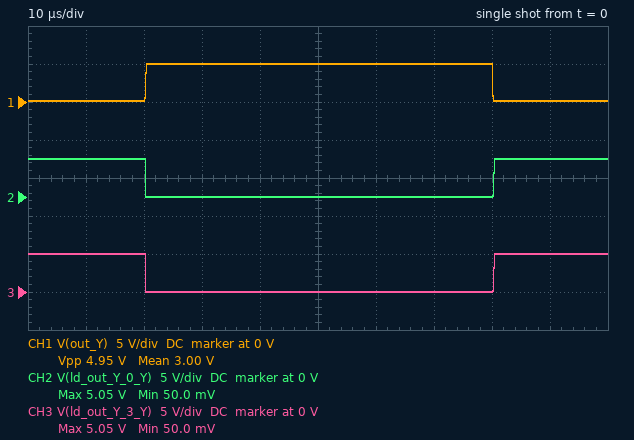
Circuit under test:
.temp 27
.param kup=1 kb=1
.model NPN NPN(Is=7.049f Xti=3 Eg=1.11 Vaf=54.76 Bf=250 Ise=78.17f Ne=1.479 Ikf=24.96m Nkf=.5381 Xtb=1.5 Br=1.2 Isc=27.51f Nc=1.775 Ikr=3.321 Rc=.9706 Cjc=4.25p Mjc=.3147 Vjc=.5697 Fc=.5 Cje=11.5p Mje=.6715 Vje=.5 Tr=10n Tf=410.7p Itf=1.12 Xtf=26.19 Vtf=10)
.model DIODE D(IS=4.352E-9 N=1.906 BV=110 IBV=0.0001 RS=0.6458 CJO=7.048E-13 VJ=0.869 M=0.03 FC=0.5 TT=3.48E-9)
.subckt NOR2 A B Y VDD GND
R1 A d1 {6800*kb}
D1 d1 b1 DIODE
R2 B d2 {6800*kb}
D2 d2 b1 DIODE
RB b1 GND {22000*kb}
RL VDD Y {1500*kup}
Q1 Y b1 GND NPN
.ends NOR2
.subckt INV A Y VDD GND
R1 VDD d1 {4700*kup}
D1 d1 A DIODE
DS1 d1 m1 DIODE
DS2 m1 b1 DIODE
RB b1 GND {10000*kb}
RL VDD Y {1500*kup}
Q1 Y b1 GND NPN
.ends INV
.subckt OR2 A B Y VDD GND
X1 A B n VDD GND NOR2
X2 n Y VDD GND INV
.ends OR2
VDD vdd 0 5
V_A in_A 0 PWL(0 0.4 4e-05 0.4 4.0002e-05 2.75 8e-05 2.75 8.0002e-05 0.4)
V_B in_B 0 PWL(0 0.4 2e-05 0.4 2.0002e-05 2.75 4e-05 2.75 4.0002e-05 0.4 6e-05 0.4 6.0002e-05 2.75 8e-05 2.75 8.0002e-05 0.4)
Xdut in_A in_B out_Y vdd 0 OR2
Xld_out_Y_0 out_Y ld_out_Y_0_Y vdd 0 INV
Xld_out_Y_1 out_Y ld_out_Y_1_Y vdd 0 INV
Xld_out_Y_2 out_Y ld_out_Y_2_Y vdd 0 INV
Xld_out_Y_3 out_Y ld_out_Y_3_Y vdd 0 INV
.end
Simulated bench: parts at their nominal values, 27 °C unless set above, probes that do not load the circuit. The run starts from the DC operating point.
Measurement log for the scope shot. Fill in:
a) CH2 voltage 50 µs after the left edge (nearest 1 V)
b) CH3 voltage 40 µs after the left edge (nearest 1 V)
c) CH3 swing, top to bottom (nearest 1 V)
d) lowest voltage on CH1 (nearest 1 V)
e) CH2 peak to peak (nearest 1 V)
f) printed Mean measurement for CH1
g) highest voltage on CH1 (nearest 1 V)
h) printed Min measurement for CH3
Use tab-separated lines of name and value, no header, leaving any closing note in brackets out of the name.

CH2 voltage 50 µs after the left edge	0 V
CH3 voltage 40 µs after the left edge	0 V
CH3 swing, top to bottom	5 V
lowest voltage on CH1	0 V
CH2 peak to peak	5 V
printed Mean measurement for CH1	3.00 V
highest voltage on CH1	5 V
printed Min measurement for CH3	50.0 mV
